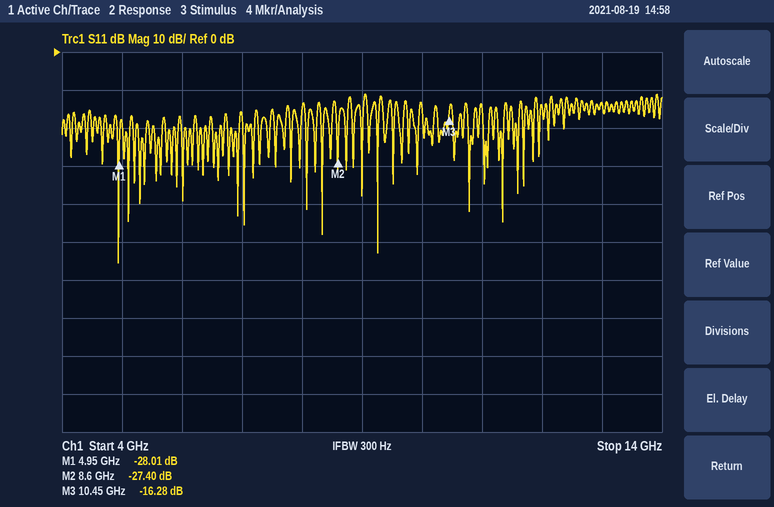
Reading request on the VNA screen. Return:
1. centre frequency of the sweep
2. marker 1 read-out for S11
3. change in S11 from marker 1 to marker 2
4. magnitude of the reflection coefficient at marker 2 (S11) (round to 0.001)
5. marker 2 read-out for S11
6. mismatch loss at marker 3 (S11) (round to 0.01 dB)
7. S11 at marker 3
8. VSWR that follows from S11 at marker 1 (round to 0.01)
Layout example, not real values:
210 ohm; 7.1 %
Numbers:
9 GHz; -28.01 dB; 0.61 dB; 0.043; -27.40 dB; 0.10 dB; -16.28 dB; 1.08
